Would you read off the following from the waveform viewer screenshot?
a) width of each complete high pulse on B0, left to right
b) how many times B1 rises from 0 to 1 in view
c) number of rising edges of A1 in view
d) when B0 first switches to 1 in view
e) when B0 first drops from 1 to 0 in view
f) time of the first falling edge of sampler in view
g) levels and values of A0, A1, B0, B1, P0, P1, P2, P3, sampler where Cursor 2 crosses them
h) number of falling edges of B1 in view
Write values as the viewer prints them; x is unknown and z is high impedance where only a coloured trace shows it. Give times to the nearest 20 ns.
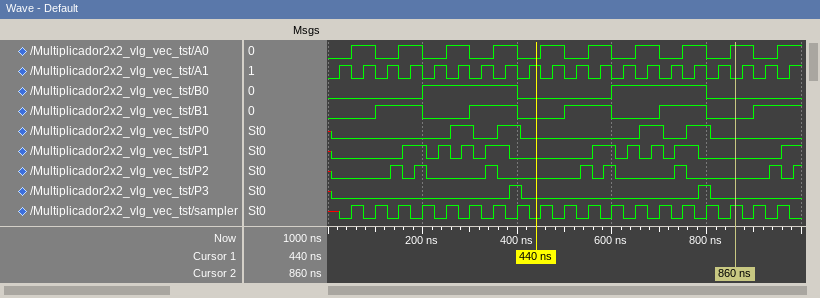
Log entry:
200 ns, 200 ns
5
20
200 ns
400 ns
80 ns
A0=1, A1=0, B0=0, B1=0, P0=0, P1=0, P2=0, P3=0, sampler=1
4
